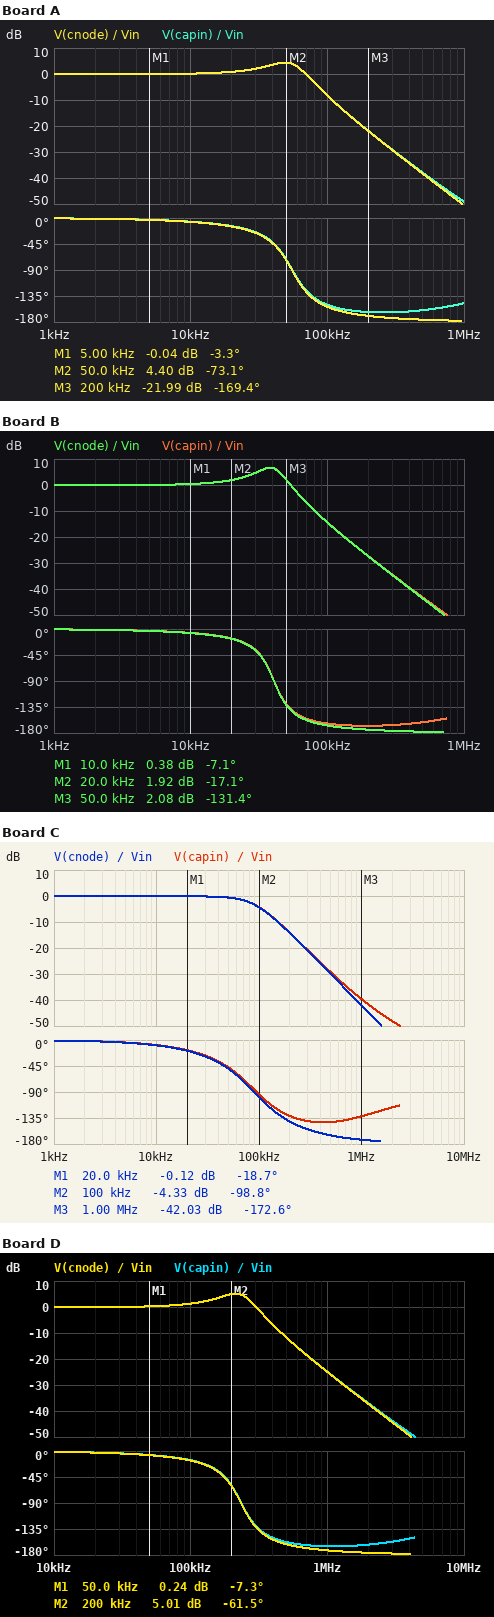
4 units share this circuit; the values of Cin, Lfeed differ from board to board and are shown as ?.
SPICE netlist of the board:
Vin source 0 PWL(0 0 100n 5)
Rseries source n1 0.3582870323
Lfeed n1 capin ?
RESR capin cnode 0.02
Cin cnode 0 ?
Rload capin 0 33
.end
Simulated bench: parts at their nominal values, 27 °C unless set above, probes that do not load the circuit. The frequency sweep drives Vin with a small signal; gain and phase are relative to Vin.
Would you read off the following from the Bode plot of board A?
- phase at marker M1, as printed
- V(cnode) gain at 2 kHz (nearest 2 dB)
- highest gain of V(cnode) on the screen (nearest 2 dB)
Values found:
-3.3 deg
0 dB
4 dB
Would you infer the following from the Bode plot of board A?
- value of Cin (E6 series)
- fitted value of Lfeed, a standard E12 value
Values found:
4.7 µF
1.8 µH
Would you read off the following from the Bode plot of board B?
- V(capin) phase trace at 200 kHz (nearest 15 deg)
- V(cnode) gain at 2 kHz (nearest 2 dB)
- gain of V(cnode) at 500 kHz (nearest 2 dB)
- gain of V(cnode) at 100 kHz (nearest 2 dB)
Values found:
-165 deg
0 dB
-44 dB
-14 dB
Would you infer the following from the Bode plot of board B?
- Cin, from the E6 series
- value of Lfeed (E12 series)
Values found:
4.7 µF
3.3 µH
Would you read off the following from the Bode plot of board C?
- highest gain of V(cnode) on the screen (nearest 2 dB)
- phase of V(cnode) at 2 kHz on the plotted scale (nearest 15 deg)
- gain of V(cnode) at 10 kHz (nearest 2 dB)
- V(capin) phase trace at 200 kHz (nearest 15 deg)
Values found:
0 dB
0 deg
0 dB
-135 deg
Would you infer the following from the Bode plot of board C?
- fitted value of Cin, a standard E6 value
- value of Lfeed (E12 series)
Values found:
6.8 µF
470 nH
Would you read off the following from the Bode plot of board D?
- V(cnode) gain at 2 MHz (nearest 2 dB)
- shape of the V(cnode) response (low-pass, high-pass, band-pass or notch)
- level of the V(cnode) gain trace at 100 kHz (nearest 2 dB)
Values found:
-38 dB
low-pass
2 dB
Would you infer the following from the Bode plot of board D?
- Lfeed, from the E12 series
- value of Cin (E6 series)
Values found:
470 nH
1 µF
